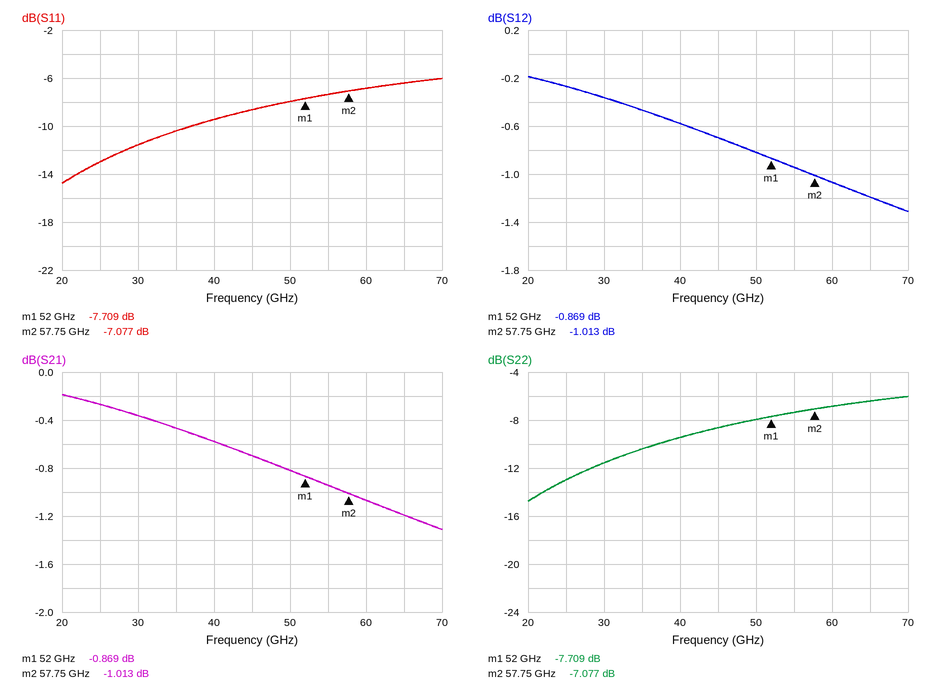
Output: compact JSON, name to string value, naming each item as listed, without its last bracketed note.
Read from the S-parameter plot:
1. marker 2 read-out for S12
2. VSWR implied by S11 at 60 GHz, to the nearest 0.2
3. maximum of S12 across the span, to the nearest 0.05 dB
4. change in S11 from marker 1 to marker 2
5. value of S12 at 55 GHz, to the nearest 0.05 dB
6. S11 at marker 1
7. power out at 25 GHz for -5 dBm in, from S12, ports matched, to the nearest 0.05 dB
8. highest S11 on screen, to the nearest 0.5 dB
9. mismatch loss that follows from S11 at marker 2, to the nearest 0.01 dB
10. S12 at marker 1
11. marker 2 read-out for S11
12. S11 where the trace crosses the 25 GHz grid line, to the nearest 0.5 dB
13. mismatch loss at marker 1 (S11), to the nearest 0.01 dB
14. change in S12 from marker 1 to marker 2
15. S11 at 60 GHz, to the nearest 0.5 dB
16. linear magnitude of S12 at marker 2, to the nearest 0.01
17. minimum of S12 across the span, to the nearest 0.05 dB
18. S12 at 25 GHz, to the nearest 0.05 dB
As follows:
{"marker 2 read-out for S12": "-1.013 dB", "VSWR implied by S11 at 60 GHz, to the nearest 0.2": "2.6", "maximum of S12 across the span, to the nearest 0.05 dB": "-0.20 dB", "change in S11 from marker 1 to marker 2": "0.632 dB", "value of S12 at 55 GHz, to the nearest 0.05 dB": "-0.95 dB", "S11 at marker 1": "-7.709 dB", "power out at 25 GHz for -5 dBm in, from S12, ports matched, to the nearest 0.05 dB": "-5.25 dBm", "highest S11 on screen, to the nearest 0.5 dB": "-6.0 dB", "mismatch loss that follows from S11 at marker 2, to the nearest 0.01 dB": "0.95 dB", "S12 at marker 1": "-0.869 dB", "marker 2 read-out for S11": "-7.077 dB", "S11 where the trace crosses the 25 GHz grid line, to the nearest 0.5 dB": "-13.0 dB", "mismatch loss at marker 1 (S11), to the nearest 0.01 dB": "0.81 dB", "change in S12 from marker 1 to marker 2": "-0.144 dB", "S11 at 60 GHz, to the nearest 0.5 dB": "-7.0 dB", "linear magnitude of S12 at marker 2, to the nearest 0.01": "0.89", "minimum of S12 across the span, to the nearest 0.05 dB": "-1.30 dB", "S12 at 25 GHz, to the nearest 0.05 dB": "-0.25 dB"}
